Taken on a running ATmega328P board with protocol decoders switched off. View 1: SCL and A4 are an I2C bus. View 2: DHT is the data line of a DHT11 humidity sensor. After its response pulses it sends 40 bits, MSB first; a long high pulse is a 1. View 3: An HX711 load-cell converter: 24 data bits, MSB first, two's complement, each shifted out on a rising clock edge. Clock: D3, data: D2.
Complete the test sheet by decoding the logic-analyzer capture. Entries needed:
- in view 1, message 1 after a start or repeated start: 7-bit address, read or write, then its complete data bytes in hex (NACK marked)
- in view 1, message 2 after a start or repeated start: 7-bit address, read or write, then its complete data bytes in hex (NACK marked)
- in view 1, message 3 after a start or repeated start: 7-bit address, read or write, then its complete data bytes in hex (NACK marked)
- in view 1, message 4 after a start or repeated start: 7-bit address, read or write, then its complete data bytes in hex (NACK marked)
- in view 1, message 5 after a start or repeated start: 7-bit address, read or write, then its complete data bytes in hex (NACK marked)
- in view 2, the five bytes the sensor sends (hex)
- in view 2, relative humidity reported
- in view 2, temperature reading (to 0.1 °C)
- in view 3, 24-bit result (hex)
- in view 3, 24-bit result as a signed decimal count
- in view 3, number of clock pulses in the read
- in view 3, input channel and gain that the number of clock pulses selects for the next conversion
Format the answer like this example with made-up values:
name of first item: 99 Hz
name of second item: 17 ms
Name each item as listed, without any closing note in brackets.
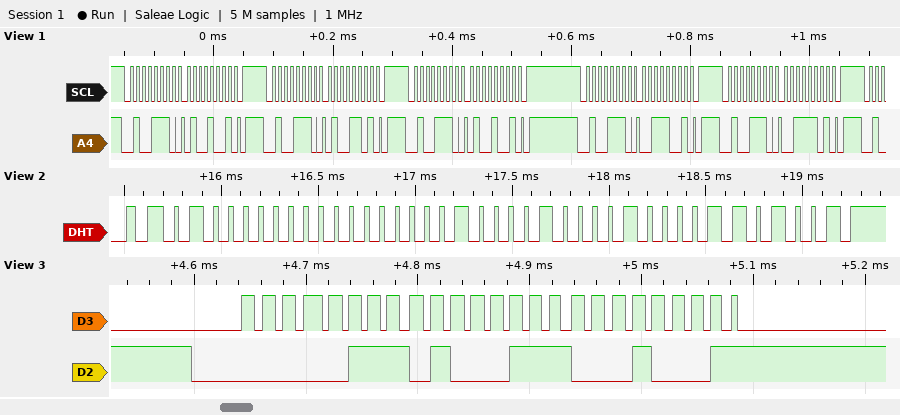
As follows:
in view 1, message 1 after a start or repeated start: 7-bit address, read or write, then its complete data bytes in hex: 0x27 write: 49
in view 1, message 2 after a start or repeated start: 7-bit address, read or write, then its complete data bytes in hex: 0x27 write: 4D
in view 1, message 3 after a start or repeated start: 7-bit address, read or write, then its complete data bytes in hex: 0x27 write: 49
in view 1, message 4 after a start or repeated start: 7-bit address, read or write, then its complete data bytes in hex: 0x27 write: 39
in view 1, message 5 after a start or repeated start: 7-bit address, read or write, then its complete data bytes in hex: 0x27 write: 3D
in view 2, the five bytes the sensor sends: 40 00 21 08 69
in view 2, relative humidity reported: 64 %
in view 2, temperature reading: 33.8 °C
in view 3, 24-bit result: 0x074711
in view 3, 24-bit result as a signed decimal count: 476945
in view 3, number of clock pulses in the read: 25
in view 3, input channel and gain that the number of clock pulses selects for the next conversion: channel A, gain 128
